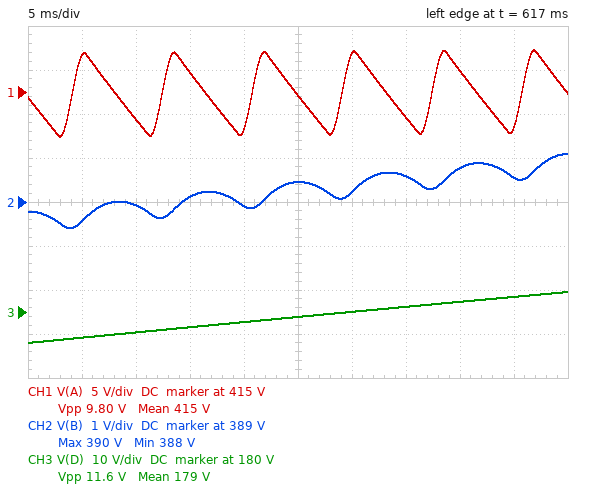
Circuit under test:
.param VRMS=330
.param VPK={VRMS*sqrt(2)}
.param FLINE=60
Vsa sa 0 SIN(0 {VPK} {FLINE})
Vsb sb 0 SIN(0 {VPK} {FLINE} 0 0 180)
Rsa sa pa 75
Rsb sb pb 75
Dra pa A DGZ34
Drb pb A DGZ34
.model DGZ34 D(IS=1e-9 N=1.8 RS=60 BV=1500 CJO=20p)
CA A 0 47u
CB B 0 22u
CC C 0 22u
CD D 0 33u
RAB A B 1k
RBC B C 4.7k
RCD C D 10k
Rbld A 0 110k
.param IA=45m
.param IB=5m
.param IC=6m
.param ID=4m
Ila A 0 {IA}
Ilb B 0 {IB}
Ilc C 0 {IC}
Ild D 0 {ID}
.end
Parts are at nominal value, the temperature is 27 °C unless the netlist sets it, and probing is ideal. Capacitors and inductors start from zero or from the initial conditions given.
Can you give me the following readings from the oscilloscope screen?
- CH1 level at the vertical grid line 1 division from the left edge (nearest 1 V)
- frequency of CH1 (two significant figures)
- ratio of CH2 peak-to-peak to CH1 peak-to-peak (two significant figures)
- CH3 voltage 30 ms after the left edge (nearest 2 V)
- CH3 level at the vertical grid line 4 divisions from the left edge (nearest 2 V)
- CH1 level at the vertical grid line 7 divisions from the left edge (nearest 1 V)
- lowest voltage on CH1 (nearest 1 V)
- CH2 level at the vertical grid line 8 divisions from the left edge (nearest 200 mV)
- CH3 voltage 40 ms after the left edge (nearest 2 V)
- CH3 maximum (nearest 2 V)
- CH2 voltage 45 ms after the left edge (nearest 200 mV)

419 V
120 Hz
0.17
180 V
178 V
412 V
410 V
389.8 V
182 V
184 V
389.6 V
